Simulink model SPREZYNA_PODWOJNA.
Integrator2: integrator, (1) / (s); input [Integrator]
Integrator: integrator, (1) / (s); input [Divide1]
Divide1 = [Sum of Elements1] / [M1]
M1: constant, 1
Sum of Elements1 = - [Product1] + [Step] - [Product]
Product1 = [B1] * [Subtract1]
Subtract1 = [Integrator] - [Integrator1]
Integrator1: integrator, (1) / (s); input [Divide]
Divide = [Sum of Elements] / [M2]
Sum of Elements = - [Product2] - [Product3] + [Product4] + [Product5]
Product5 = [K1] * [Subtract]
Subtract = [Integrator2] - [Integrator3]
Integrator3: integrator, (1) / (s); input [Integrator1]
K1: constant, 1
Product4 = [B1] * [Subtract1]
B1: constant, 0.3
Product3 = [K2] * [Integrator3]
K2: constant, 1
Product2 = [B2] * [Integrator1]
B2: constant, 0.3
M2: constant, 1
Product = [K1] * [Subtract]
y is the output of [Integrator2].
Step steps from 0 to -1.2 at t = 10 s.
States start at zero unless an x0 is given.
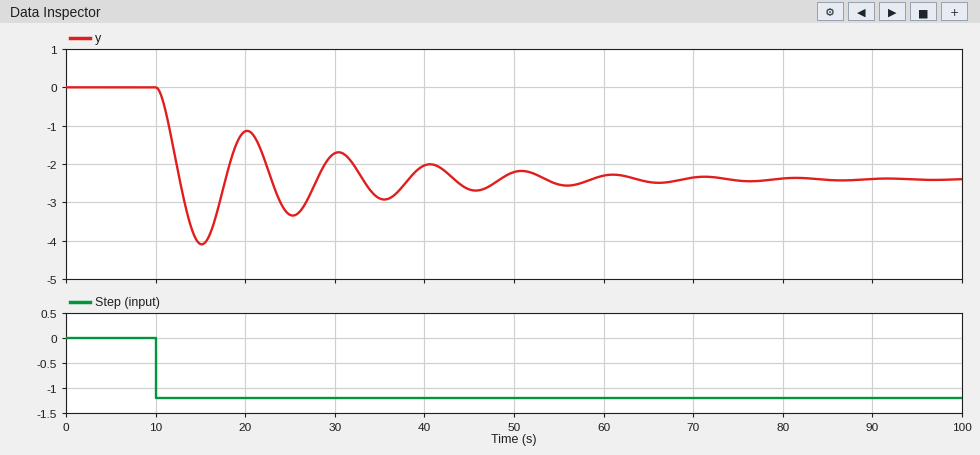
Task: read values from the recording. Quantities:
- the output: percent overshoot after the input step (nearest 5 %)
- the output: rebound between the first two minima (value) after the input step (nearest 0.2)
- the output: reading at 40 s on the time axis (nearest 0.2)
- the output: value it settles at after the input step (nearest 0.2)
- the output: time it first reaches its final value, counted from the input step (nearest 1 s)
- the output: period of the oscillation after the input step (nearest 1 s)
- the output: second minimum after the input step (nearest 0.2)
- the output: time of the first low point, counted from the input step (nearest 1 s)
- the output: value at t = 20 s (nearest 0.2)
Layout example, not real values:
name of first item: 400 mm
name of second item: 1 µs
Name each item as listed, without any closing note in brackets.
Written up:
the output: percent overshoot after the input step: 70 %
the output: rebound between the first two minima (value) after the input step: -1.2
the output: reading at 40 s on the time axis: -2.0
the output: value it settles at after the input step: -2.4
the output: time it first reaches its final value, counted from the input step: 3 s
the output: period of the oscillation after the input step: 10 s
the output: second minimum after the input step: -3.4
the output: time of the first low point, counted from the input step: 5 s
the output: value at t = 20 s: -1.2
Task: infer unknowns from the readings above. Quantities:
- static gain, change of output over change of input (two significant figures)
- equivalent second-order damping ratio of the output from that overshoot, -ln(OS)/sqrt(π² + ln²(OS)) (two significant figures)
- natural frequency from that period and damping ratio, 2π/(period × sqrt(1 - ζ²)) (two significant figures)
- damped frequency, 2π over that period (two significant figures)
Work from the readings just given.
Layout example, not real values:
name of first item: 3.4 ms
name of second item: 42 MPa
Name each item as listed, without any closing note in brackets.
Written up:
static gain, change of output over change of input: 2.0
equivalent second-order damping ratio of the output from that overshoot, -ln(OS)/sqrt(π² + ln²(OS)): 0.11
natural frequency from that period and damping ratio, 2π/(period × sqrt(1 - ζ²)): 0.63 rad/s
damped frequency, 2π over that period: 0.63 rad/s
